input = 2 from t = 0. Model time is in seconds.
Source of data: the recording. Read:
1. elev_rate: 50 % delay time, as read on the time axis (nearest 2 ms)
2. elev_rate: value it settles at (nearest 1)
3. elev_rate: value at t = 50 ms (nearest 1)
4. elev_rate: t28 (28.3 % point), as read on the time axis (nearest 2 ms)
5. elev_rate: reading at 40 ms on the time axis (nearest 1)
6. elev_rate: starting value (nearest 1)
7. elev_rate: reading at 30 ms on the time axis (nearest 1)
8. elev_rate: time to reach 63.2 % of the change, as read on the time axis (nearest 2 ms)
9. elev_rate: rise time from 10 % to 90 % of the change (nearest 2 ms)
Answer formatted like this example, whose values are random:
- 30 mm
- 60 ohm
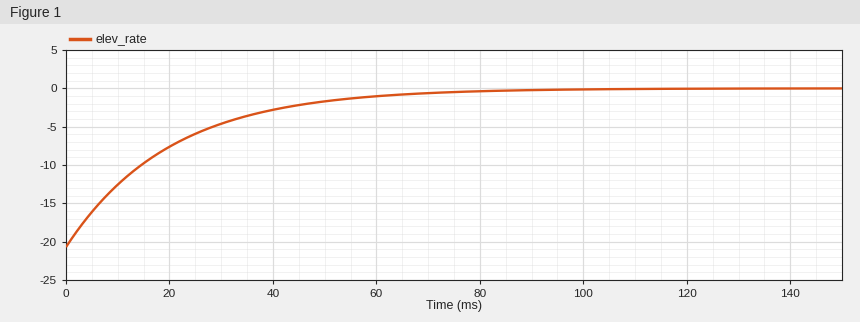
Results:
- 14 ms
- 0
- -2
- 6 ms
- -3
- -21
- -5
- 20 ms
- 44 ms
